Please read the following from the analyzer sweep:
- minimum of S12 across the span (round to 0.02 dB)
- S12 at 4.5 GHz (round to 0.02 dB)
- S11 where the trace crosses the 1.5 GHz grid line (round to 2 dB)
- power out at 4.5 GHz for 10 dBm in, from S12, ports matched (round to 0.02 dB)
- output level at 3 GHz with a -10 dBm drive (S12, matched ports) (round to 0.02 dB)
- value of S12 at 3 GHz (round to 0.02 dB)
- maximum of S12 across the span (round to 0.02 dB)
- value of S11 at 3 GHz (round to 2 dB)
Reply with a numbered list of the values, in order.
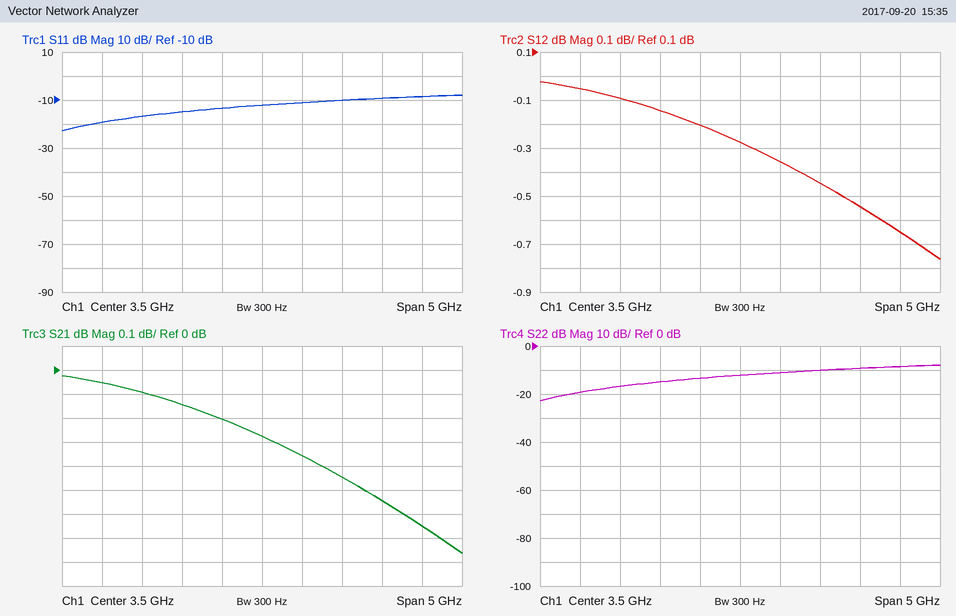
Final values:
1. -0.76 dB
2. -0.44 dB
3. -20 dB
4. 9.56 dBm
5. -10.20 dBm
6. -0.20 dB
7. -0.02 dB
8. -14 dB
